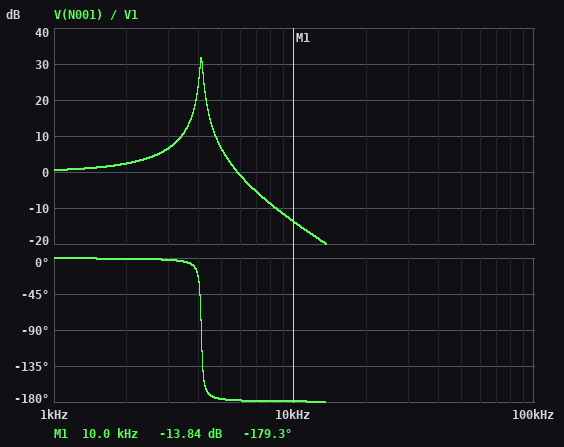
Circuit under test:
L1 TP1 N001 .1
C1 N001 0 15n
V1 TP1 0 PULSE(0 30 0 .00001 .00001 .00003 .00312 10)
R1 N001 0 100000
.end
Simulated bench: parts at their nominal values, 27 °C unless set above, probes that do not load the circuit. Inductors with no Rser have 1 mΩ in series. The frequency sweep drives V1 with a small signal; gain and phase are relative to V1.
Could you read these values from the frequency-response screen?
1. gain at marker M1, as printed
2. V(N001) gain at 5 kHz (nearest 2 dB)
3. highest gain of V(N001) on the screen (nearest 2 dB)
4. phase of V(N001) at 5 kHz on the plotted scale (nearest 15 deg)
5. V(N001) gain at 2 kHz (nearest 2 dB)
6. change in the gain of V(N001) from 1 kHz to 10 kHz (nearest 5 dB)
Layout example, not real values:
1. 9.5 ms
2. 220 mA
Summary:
1. -13.84 dB
2. 6 dB
3. 32 dB
4. -180 deg
5. 2 dB
6. -15 dB
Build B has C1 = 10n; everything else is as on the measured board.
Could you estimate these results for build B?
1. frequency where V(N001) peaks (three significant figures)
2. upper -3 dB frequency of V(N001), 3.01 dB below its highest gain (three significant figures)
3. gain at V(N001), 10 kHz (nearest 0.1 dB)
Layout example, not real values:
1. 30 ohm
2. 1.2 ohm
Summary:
1. 5.03 kHz
2. 5.11 kHz
3. -9.4 dB
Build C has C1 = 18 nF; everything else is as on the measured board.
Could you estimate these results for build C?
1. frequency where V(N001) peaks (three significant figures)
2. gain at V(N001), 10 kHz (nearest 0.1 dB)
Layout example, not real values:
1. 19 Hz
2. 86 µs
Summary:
1. 3.75 kHz
2. -15.7 dB
